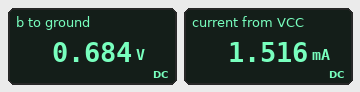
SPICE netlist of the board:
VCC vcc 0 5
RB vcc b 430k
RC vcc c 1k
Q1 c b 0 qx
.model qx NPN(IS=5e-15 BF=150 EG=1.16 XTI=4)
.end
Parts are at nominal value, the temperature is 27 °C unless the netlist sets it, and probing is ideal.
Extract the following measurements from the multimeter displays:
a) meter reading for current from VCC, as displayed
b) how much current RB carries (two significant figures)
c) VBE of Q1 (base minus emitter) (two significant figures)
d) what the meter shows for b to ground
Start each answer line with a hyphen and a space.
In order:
- 1.516 mA
- 10 µA
- 680 mV
- 0.684 V
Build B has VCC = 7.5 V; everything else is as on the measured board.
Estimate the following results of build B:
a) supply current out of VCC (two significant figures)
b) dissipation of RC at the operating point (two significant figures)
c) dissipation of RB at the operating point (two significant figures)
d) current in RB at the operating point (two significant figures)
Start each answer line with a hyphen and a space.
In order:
- 2.4 mA
- 5.6 mW
- 110 µW
- 16 µA
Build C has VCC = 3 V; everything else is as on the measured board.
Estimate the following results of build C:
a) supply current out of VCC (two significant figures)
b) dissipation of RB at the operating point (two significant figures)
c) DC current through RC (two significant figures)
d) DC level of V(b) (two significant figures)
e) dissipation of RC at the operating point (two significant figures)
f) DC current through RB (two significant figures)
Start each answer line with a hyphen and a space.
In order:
- 820 µA
- 13 µW
- 810 µA
- 670 mV
- 660 µW
- 5.4 µA
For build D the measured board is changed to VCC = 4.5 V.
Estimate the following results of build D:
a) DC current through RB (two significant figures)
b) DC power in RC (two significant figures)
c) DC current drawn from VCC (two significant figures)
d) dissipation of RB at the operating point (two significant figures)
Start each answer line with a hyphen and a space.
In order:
- 8.9 µA
- 1.8 mW
- 1.3 mA
- 34 µW
